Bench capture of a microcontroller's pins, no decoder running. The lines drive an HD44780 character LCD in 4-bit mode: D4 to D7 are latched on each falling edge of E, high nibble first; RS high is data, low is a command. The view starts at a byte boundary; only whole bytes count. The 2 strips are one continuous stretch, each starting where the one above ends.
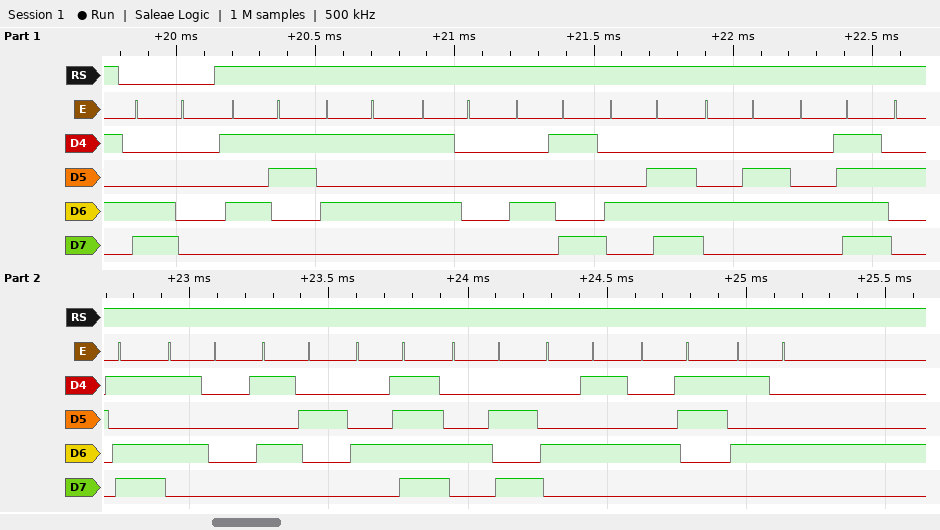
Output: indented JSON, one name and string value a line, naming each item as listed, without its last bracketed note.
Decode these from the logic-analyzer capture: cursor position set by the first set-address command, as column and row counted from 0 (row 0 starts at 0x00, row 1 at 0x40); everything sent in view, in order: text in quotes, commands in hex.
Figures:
{
  "cursor position set by the first set-address command, as column and row counted from 0": "column 0, row 1",
  "everything sent in view, in order: text in quotes, commands in hex": "0xC0 \"SUPINFO-PROJECT\""
}
